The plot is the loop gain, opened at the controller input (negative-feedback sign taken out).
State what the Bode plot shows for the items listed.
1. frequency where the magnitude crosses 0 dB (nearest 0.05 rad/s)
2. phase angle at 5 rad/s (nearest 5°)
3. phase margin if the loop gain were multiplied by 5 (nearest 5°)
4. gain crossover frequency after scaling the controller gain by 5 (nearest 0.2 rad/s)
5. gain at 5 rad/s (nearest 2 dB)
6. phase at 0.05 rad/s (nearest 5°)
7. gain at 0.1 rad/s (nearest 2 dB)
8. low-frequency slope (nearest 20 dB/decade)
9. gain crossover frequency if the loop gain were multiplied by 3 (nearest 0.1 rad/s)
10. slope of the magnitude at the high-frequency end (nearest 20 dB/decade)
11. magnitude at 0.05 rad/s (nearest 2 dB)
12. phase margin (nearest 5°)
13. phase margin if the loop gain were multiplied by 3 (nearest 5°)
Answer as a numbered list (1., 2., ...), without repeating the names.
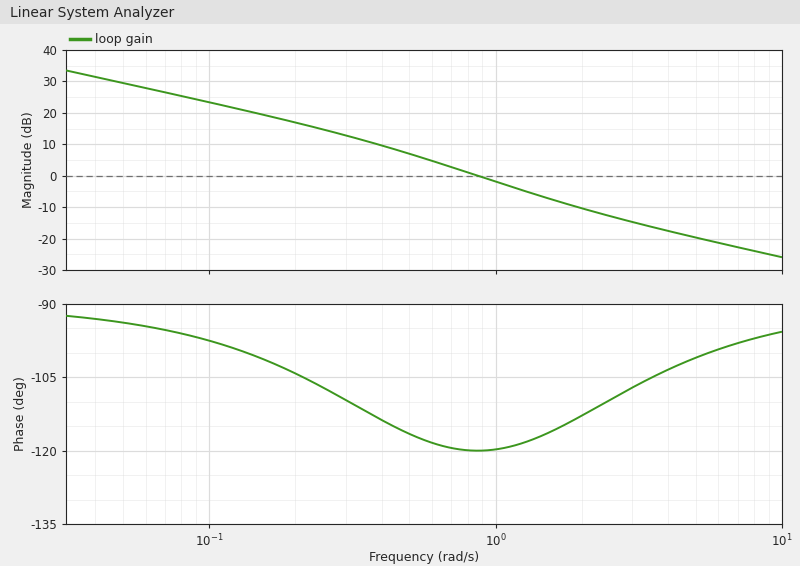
1. 0.85 rad/s
2. -100°
3. 70°
4. 2.8 rad/s
5. -20 dB
6. -95°
7. 24 dB
8. -20 dB/decade
9. 1.9 rad/s
10. -20 dB/decade
11. 30 dB
12. 60°
13. 65°
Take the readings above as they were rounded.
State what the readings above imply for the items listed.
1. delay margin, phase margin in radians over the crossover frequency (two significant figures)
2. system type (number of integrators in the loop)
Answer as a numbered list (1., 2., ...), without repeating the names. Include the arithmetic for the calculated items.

1. 60 × π / 180 / 0.85 = 1.2 s
2. 1
